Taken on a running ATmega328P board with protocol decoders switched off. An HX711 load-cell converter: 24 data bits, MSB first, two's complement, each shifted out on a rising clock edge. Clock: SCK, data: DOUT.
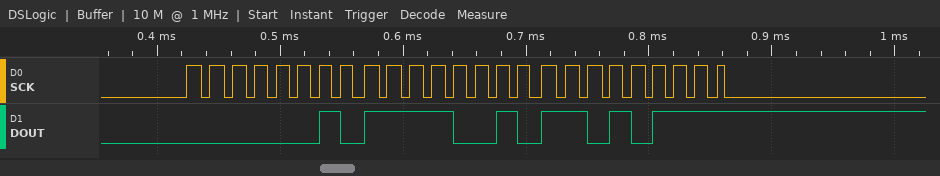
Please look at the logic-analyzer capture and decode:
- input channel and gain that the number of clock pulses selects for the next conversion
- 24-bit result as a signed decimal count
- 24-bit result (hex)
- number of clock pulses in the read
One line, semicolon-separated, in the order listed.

channel A, gain 128; 193239; 0x02F2D7; 25
